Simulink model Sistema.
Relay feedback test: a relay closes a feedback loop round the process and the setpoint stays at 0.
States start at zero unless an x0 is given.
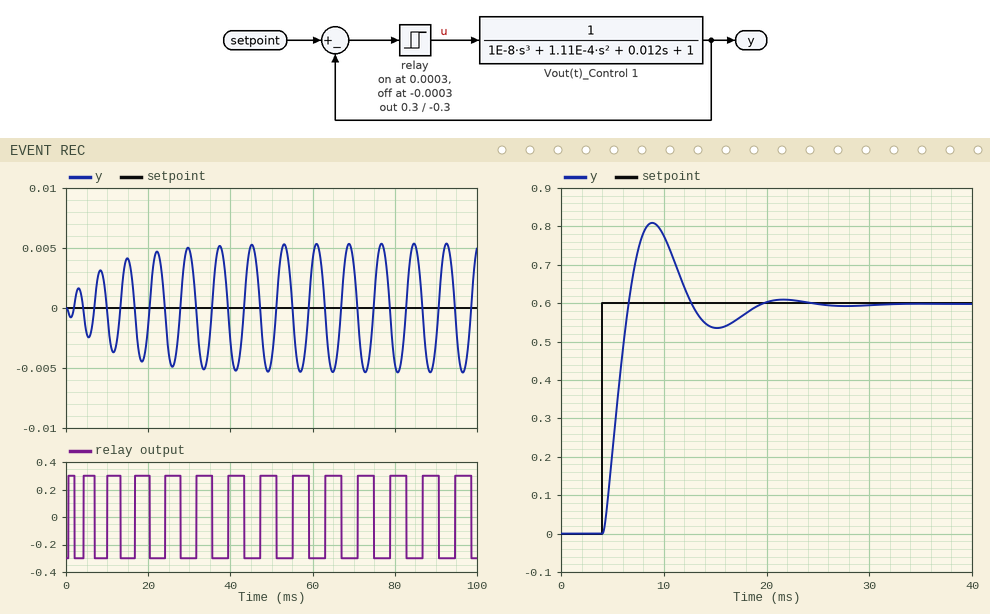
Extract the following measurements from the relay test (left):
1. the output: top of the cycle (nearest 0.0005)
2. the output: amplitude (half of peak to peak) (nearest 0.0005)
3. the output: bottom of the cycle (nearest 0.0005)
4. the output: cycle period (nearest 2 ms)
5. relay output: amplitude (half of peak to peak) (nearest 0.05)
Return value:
0.0055
0.0055
-0.0055
8 ms
0.30
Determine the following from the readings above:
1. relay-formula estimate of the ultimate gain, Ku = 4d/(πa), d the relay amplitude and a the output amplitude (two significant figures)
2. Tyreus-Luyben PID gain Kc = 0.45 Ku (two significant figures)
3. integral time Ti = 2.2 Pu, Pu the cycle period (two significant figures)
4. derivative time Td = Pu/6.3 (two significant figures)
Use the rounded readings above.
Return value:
69
31
18 ms
1.3 ms
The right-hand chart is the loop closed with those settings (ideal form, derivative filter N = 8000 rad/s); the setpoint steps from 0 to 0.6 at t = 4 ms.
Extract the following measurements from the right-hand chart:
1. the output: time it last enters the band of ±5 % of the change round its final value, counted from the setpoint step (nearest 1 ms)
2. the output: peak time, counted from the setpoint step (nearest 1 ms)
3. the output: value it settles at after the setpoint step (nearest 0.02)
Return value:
14 ms
5 ms
0.60
